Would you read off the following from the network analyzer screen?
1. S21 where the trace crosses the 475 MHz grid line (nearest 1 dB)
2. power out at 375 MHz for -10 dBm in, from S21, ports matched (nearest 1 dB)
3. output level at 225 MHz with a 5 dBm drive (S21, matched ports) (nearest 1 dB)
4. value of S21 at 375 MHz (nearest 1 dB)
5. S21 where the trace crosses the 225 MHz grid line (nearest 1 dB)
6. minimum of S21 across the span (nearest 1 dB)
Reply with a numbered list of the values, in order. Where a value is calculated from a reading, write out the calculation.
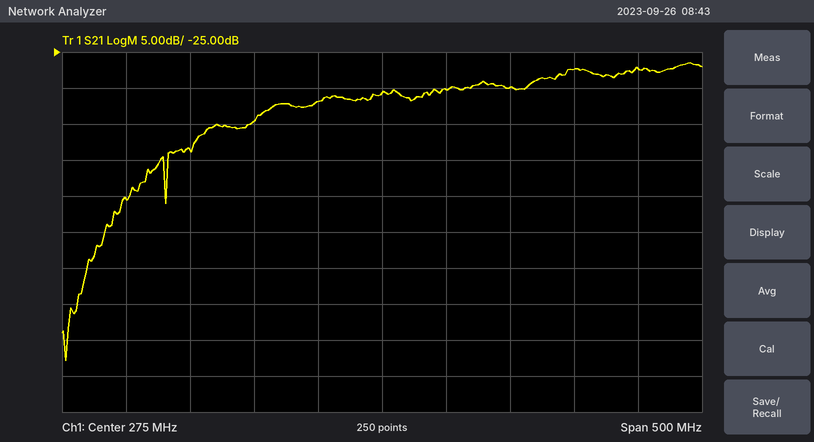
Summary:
1. -27 dB
2. -10 dBm + (-30 dB) = -40 dBm
3. 5 dBm + (-32 dB) = -27 dBm
4. -30 dB
5. -32 dB
6. -68 dB
